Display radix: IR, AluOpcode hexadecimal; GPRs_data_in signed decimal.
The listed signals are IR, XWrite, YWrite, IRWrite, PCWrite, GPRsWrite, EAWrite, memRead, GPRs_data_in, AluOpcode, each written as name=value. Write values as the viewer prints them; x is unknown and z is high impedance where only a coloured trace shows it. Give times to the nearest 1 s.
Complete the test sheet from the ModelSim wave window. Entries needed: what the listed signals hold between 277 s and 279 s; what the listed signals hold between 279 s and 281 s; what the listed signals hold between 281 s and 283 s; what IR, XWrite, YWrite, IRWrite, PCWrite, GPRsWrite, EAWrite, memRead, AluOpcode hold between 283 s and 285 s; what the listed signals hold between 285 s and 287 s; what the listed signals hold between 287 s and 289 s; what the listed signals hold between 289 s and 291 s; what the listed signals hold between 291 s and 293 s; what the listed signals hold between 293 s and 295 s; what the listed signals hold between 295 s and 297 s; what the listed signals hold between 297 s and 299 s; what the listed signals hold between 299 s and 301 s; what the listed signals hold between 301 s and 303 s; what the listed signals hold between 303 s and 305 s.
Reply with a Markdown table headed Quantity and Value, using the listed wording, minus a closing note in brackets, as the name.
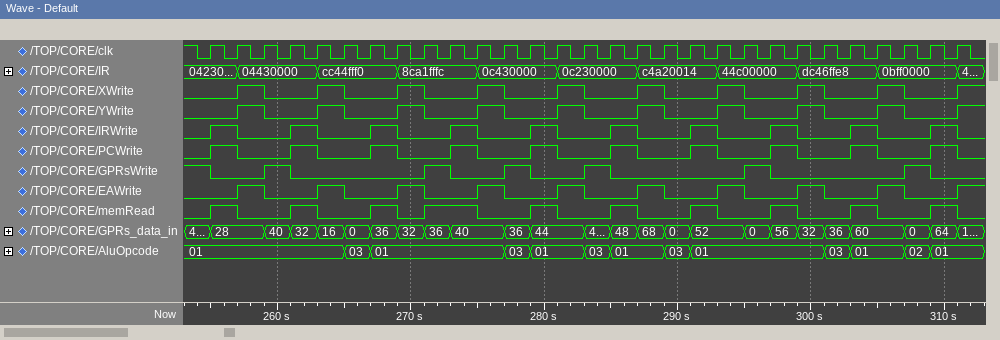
| Quantity | Value |
|---|---|
| what the listed signals hold between 277 s and 279 s | IR=0c430000, XWrite=0, YWrite=0, IRWrite=0, PCWrite=0, GPRsWrite=1, EAWrite=0, memRead=0, GPRs_data_in=36, AluOpcode=03 |
| what the listed signals hold between 279 s and 281 s | IR=0c430000, XWrite=0, YWrite=0, IRWrite=1, PCWrite=1, GPRsWrite=0, EAWrite=0, memRead=1, GPRs_data_in=44, AluOpcode=01 |
| what the listed signals hold between 281 s and 283 s | IR=0c230000, XWrite=1, YWrite=1, IRWrite=0, PCWrite=0, GPRsWrite=0, EAWrite=1, memRead=0, GPRs_data_in=44, AluOpcode=01 |
| what IR, XWrite, YWrite, IRWrite, PCWrite, GPRsWrite, EAWrite, memRead, AluOpcode hold between 283 s and 285 s | IR=0c230000, XWrite=0, YWrite=0, IRWrite=0, PCWrite=0, GPRsWrite=1, EAWrite=0, memRead=0, AluOpcode=03 |
| what the listed signals hold between 285 s and 287 s | IR=0c230000, XWrite=0, YWrite=0, IRWrite=1, PCWrite=1, GPRsWrite=0, EAWrite=0, memRead=1, GPRs_data_in=48, AluOpcode=01 |
| what the listed signals hold between 287 s and 289 s | IR=c4a20014, XWrite=1, YWrite=1, IRWrite=0, PCWrite=0, GPRsWrite=0, EAWrite=1, memRead=0, GPRs_data_in=68, AluOpcode=01 |
| what the listed signals hold between 289 s and 291 s | IR=c4a20014, XWrite=0, YWrite=0, IRWrite=0, PCWrite=0, GPRsWrite=0, EAWrite=0, memRead=0, GPRs_data_in=0, AluOpcode=03 |
| what the listed signals hold between 291 s and 293 s | IR=c4a20014, XWrite=0, YWrite=0, IRWrite=1, PCWrite=1, GPRsWrite=0, EAWrite=0, memRead=1, GPRs_data_in=52, AluOpcode=01 |
| what the listed signals hold between 293 s and 295 s | IR=44c00000, XWrite=1, YWrite=1, IRWrite=0, PCWrite=0, GPRsWrite=0, EAWrite=1, memRead=0, GPRs_data_in=52, AluOpcode=01 |
| what the listed signals hold between 295 s and 297 s | IR=44c00000, XWrite=0, YWrite=0, IRWrite=0, PCWrite=0, GPRsWrite=1, EAWrite=0, memRead=0, GPRs_data_in=0, AluOpcode=01 |
| what the listed signals hold between 297 s and 299 s | IR=44c00000, XWrite=0, YWrite=0, IRWrite=1, PCWrite=1, GPRsWrite=0, EAWrite=0, memRead=1, GPRs_data_in=56, AluOpcode=01 |
| what the listed signals hold between 299 s and 301 s | IR=dc46ffe8, XWrite=1, YWrite=1, IRWrite=0, PCWrite=0, GPRsWrite=0, EAWrite=1, memRead=0, GPRs_data_in=32, AluOpcode=01 |
| what the listed signals hold between 301 s and 303 s | IR=dc46ffe8, XWrite=0, YWrite=0, IRWrite=0, PCWrite=0, GPRsWrite=0, EAWrite=0, memRead=0, GPRs_data_in=36, AluOpcode=03 |
| what the listed signals hold between 303 s and 305 s | IR=dc46ffe8, XWrite=0, YWrite=0, IRWrite=1, PCWrite=1, GPRsWrite=0, EAWrite=0, memRead=1, GPRs_data_in=60, AluOpcode=01 |
